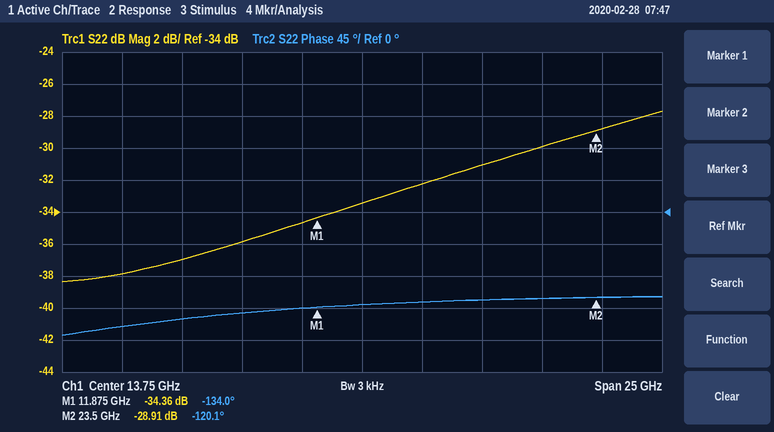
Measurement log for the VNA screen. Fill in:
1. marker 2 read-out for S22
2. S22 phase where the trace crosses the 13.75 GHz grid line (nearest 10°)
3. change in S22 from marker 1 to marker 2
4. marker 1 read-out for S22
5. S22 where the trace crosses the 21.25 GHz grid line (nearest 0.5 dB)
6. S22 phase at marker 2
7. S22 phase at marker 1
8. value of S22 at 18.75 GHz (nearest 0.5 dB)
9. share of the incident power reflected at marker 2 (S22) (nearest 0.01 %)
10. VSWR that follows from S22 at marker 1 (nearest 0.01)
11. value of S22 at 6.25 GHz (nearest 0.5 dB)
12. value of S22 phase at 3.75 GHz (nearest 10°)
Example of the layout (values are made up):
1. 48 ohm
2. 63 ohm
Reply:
1. -28.91 dB
2. -130°
3. 5.45 dB
4. -34.36 dB
5. -30.0 dB
6. -120.1°
7. -134.0°
8. -31.0 dB
9. 0.13 %
10. 1.04
11. -37.0 dB
12. -160°
